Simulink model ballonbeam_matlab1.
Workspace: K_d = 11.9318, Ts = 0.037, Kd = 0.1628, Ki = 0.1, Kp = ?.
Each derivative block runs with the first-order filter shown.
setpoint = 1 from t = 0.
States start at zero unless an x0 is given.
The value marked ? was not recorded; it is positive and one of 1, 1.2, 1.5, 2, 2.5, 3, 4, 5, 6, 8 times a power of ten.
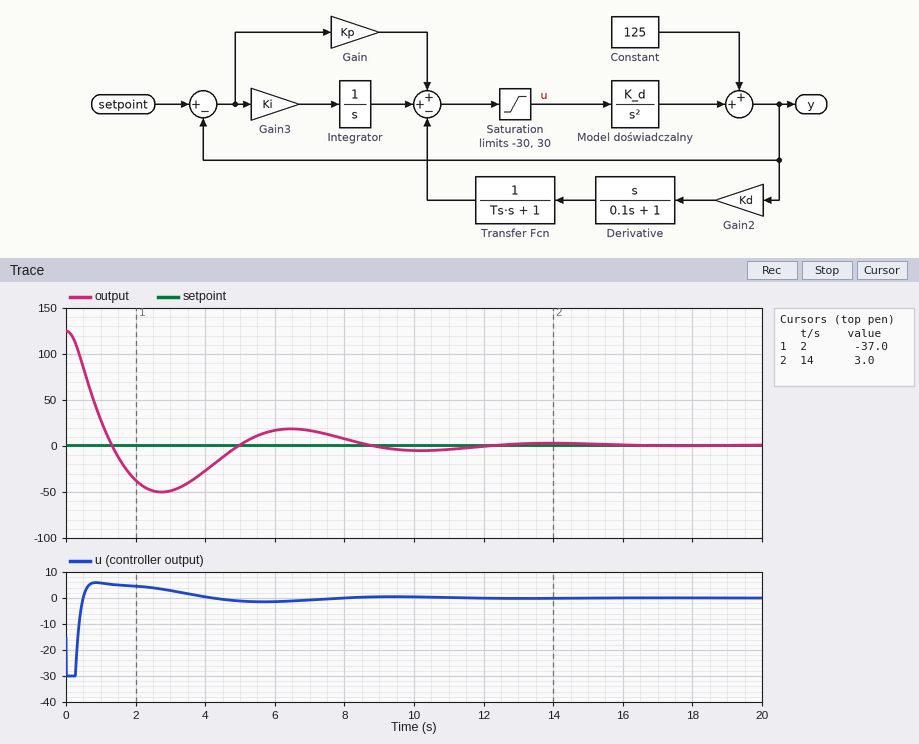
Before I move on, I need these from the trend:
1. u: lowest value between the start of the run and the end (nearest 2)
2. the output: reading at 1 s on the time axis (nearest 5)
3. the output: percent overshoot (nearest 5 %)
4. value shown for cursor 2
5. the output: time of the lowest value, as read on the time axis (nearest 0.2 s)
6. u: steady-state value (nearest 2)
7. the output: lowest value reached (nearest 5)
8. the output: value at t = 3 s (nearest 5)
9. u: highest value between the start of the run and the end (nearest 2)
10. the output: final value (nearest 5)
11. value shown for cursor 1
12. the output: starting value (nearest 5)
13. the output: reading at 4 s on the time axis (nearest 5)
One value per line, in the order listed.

-30
30
40 %
3.0
2.8 s
0
-50
-50
6
0
-37.0
125
-25
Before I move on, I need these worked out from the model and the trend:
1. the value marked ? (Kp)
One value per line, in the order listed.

0.12
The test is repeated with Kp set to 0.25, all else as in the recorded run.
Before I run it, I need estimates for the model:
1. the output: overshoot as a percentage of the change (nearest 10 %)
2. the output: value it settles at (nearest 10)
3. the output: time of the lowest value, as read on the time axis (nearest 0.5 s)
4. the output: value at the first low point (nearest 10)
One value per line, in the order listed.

30 %
0
2.0 s
-40
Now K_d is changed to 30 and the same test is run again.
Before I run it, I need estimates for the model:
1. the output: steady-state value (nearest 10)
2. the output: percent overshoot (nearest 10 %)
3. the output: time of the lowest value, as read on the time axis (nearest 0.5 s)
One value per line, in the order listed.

0
20 %
3.0 s
